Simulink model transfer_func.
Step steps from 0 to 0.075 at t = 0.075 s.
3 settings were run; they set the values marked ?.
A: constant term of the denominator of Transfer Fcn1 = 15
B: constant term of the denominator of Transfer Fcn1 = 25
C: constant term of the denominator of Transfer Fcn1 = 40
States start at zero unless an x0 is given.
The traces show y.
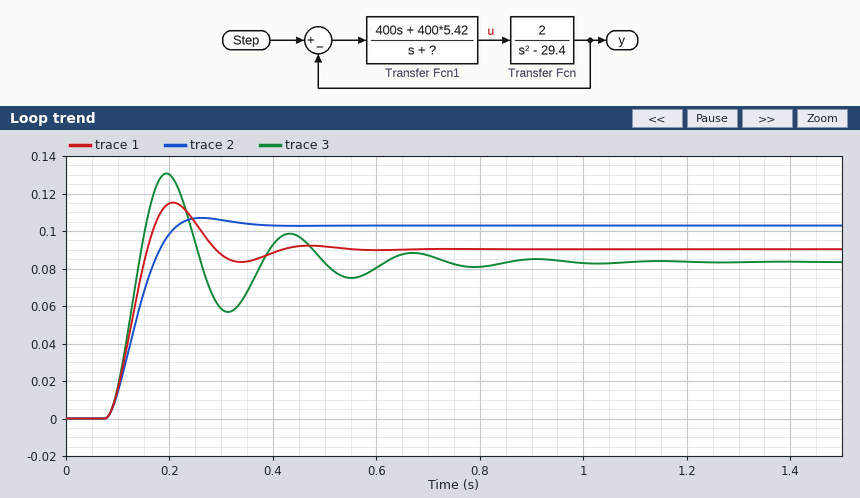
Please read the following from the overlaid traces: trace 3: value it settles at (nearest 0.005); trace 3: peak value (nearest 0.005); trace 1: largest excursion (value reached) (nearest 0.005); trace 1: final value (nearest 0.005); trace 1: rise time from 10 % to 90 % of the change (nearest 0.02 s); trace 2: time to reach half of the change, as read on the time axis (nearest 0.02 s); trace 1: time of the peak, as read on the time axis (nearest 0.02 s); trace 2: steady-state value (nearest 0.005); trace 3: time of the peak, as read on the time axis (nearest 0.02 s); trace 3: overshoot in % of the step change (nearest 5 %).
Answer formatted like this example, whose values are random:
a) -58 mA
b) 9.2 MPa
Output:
a) 0.085
b) 0.130
c) 0.115
d) 0.090
e) 0.06 s
f) 0.14 s
g) 0.20 s
h) 0.105
i) 0.20 s
j) 55 %
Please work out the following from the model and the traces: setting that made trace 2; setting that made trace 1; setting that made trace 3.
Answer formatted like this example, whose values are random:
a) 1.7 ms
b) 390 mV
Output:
a) C
b) B
c) A
